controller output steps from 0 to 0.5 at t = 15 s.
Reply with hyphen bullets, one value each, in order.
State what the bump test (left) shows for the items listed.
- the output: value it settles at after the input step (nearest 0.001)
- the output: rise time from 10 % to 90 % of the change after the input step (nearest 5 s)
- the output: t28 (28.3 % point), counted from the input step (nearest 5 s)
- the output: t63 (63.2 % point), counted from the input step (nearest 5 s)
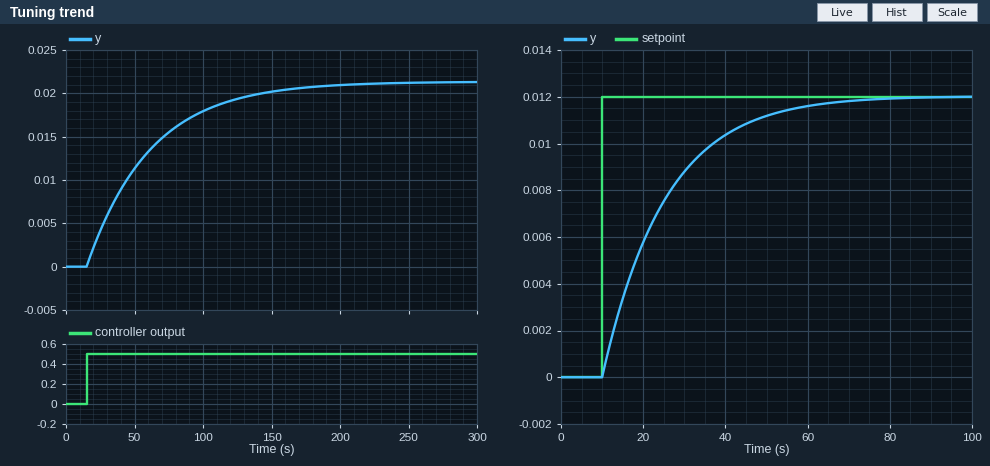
- 0.021
- 100 s
- 15 s
- 45 s
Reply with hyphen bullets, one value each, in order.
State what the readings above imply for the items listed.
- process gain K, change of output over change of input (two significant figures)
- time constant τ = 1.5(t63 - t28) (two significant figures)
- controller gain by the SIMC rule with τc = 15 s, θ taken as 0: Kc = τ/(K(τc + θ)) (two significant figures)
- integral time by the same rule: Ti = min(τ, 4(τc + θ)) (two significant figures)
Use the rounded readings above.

- 0.042
- 45 s
- 71
- 45 s
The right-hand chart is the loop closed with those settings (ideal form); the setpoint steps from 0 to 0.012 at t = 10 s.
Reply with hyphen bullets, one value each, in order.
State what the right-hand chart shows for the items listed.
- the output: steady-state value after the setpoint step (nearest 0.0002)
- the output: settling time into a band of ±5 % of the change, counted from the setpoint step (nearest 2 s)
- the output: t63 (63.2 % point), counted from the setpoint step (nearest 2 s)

- 0.0120
- 44 s
- 16 s
